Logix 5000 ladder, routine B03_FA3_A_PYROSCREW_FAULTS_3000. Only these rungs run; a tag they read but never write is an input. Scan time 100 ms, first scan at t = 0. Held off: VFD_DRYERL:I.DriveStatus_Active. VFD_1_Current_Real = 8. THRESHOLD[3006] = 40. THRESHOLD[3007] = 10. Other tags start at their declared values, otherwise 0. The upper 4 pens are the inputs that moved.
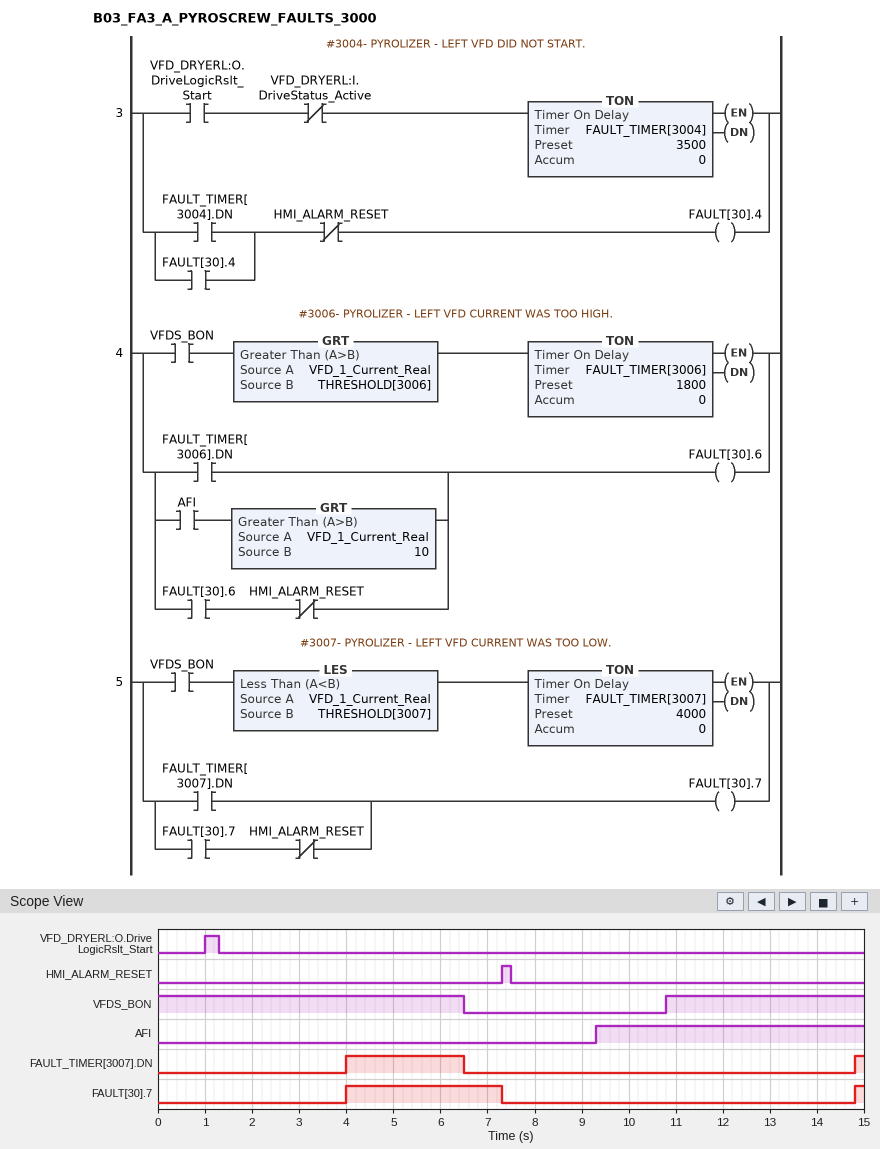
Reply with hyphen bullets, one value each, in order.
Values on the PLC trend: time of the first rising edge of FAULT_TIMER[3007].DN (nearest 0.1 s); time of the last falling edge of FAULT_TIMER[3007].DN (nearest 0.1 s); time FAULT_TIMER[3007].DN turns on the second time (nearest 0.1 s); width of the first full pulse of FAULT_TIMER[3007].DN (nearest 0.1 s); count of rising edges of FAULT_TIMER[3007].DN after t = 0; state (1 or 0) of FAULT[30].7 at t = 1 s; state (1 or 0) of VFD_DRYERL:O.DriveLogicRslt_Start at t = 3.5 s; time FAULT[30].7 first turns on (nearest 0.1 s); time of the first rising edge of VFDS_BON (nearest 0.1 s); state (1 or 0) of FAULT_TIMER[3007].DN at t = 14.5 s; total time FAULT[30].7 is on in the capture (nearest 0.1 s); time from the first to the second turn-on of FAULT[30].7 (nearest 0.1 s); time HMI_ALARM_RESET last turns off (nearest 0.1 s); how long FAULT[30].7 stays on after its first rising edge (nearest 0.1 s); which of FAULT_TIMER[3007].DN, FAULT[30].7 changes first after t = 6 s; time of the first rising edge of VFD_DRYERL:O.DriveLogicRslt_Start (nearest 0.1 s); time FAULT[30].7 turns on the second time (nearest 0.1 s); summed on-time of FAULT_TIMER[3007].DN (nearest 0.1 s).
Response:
- 4.0 s
- 6.5 s
- 14.8 s
- 2.5 s
- 2
- 0
- 0
- 4.0 s
- 10.8 s
- 0
- 3.5 s
- 10.8 s
- 7.5 s
- 3.3 s
- FAULT_TIMER[3007].DN
- 1.0 s
- 14.8 s
- 2.7 s
